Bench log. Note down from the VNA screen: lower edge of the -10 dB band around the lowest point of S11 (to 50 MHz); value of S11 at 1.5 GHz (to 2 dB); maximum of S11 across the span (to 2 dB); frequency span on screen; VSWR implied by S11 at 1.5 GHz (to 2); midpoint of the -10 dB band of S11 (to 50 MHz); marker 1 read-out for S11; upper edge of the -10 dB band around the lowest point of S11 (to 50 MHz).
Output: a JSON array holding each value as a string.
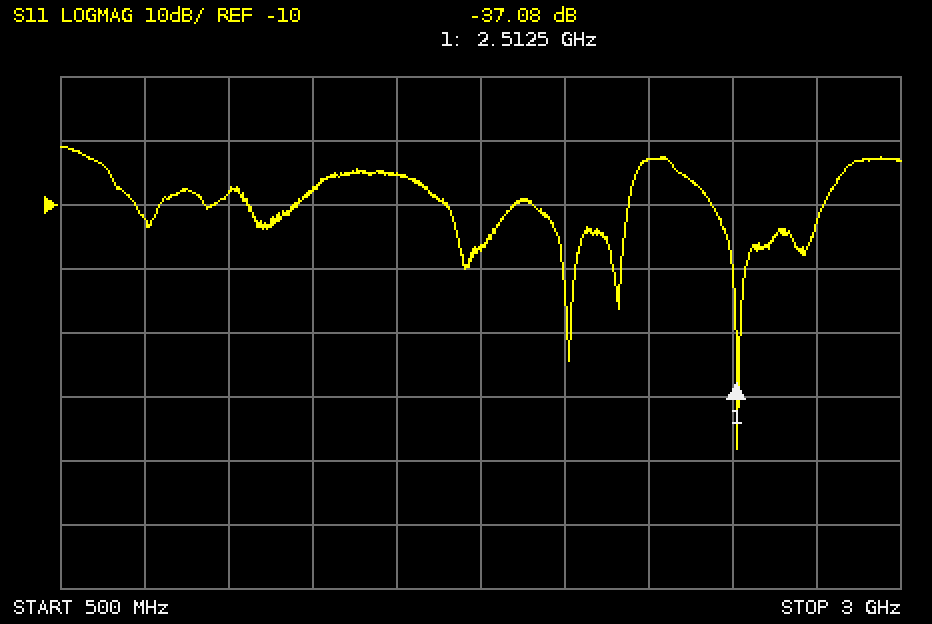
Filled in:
["2.45 GHz", "-6 dB", "0 dB", "2.5 GHz", "4", "2.60 GHz", "-37.08 dB", "2.75 GHz"]
